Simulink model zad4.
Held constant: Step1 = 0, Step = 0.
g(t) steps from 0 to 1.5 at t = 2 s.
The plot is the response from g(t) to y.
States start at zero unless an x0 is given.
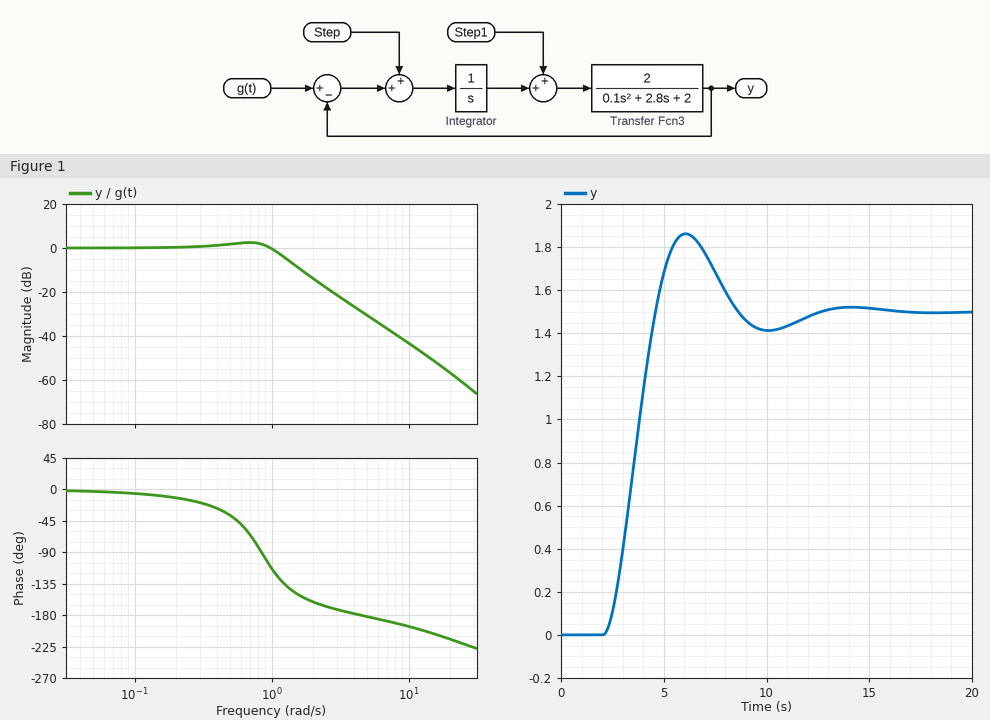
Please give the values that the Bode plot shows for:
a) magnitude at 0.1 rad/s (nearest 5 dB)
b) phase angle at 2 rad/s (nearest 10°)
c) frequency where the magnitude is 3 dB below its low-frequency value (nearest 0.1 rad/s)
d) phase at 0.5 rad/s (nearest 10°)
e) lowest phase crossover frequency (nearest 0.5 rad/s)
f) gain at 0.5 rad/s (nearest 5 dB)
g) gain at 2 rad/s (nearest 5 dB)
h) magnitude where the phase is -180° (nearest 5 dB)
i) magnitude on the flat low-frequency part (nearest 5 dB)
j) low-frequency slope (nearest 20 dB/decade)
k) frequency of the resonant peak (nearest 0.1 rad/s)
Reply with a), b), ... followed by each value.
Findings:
a) 0 dB
b) -160°
c) 1.2 rad/s
d) -40°
e) 4.5 rad/s
f) 0 dB
g) -15 dB
h) -30 dB
i) 0 dB
j) 0 dB/decade
k) 0.7 rad/s
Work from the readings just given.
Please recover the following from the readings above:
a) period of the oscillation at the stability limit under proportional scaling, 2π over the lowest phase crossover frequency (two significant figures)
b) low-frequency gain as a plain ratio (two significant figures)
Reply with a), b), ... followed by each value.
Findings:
a) 1.4 s
b) 1.0
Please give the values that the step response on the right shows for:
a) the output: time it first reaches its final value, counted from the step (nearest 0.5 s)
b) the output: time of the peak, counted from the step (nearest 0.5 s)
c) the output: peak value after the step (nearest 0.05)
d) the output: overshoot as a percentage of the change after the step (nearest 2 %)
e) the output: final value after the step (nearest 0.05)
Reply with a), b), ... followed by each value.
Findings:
a) 2.5 s
b) 4.0 s
c) 1.85
d) 24 %
e) 1.50
